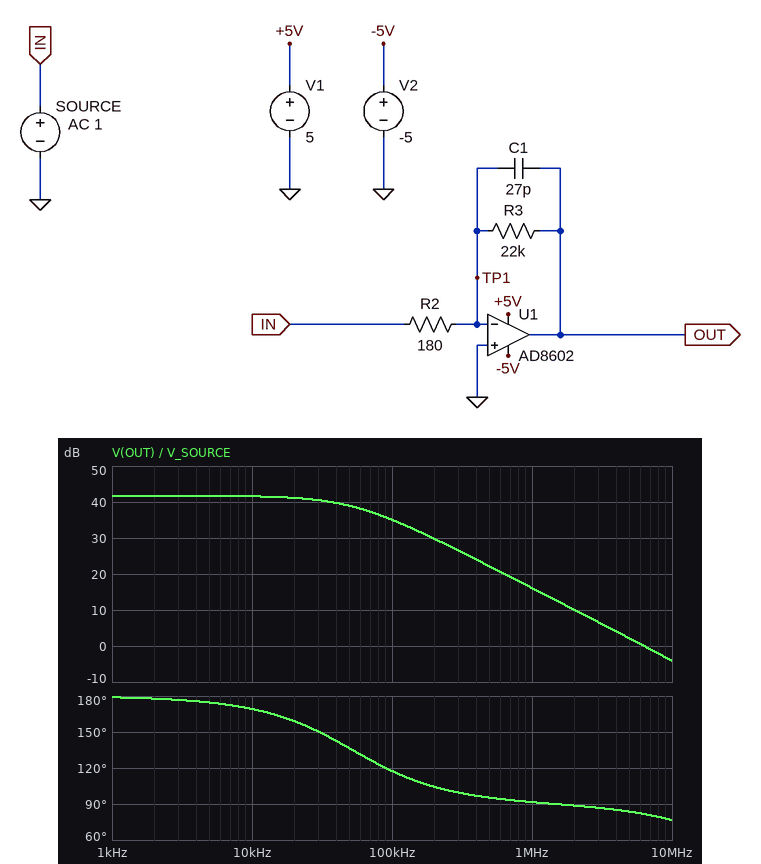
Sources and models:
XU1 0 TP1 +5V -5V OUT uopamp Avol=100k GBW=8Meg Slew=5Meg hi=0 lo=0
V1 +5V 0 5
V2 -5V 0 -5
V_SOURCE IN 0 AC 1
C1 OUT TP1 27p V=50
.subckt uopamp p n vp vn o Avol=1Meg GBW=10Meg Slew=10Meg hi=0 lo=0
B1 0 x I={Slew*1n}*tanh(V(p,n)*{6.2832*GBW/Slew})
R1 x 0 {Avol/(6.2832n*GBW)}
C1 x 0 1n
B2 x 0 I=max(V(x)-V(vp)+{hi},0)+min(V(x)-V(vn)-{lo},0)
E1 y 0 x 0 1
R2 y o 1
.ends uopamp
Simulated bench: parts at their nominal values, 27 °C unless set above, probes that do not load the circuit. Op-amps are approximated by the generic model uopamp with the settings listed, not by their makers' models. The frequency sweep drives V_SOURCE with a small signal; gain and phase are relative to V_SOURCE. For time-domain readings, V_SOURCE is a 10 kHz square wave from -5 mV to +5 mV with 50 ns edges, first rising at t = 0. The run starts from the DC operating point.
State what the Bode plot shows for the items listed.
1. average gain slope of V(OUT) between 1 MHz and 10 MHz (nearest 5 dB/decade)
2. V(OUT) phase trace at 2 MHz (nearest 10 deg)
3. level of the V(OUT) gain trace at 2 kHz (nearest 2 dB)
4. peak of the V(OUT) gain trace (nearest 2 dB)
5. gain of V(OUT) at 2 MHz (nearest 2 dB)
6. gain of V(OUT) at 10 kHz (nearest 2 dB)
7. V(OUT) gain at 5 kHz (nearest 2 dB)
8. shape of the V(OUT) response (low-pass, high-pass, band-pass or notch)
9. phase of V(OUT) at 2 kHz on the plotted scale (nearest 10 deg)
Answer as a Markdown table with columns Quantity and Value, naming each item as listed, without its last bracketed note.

| Quantity | Value |
|---|---|
| average gain slope of V(OUT) between 1 MHz and 10 MHz | -20 dB/decade |
| V(OUT) phase trace at 2 MHz | 90 deg |
| level of the V(OUT) gain trace at 2 kHz | 42 dB |
| peak of the V(OUT) gain trace | 42 dB |
| gain of V(OUT) at 2 MHz | 10 dB |
| gain of V(OUT) at 10 kHz | 42 dB |
| V(OUT) gain at 5 kHz | 42 dB |
| shape of the V(OUT) response | low-pass |
| phase of V(OUT) at 2 kHz on the plotted scale | 180 deg |
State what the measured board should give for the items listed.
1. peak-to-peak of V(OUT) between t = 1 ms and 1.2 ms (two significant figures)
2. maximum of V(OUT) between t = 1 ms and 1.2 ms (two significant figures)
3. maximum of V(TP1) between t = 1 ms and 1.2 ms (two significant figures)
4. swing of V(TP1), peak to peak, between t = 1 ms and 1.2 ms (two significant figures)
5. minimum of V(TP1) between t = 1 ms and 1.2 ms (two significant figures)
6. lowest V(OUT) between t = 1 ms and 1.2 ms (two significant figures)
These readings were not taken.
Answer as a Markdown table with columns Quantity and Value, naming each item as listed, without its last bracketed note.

| Quantity | Value |
|---|---|
| peak-to-peak of V(OUT) between t = 1 ms and 1.2 ms | 1.2 V |
| maximum of V(OUT) between t = 1 ms and 1.2 ms | 610 mV |
| maximum of V(TP1) between t = 1 ms and 1.2 ms | 7.9 mV |
| swing of V(TP1), peak to peak, between t = 1 ms and 1.2 ms | 16 mV |
| minimum of V(TP1) between t = 1 ms and 1.2 ms | -7.9 mV |
| lowest V(OUT) between t = 1 ms and 1.2 ms | -610 mV |
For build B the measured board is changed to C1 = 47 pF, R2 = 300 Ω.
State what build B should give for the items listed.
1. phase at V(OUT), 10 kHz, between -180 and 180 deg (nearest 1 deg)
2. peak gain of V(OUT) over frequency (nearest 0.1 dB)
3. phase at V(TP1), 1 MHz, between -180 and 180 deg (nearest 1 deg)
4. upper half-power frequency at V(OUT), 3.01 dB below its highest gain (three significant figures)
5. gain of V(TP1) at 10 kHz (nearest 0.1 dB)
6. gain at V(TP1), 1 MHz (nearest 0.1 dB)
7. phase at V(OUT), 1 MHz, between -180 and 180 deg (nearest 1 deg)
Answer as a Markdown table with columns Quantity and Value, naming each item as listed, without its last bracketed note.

| Quantity | Value |
|---|---|
| phase at V(OUT), 10 kHz, between -180 and 180 deg | 171 deg |
| peak gain of V(OUT) over frequency | 37.3 dB |
| phase at V(TP1), 1 MHz, between -180 and 180 deg | 1 deg |
| upper half-power frequency at V(OUT), 3.01 dB below its highest gain | 63.6 kHz |
| gain of V(TP1) at 10 kHz | -20.9 dB |
| gain at V(TP1), 1 MHz | -4.7 dB |
| phase at V(OUT), 1 MHz, between -180 and 180 deg | 91 deg |
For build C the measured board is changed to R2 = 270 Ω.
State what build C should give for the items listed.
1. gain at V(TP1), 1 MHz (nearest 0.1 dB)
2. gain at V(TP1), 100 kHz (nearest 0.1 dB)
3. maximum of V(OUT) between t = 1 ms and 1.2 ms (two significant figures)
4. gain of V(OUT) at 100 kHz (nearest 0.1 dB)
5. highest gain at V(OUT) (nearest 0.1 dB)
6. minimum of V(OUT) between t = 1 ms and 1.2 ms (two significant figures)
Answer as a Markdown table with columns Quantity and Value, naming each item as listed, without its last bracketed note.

| Quantity | Value |
|---|---|
| gain at V(TP1), 1 MHz | -2.8 dB |
| gain at V(TP1), 100 kHz | -4.6 dB |
| maximum of V(OUT) between t = 1 ms and 1.2 ms | 410 mV |
| gain of V(OUT) at 100 kHz | 33.5 dB |
| highest gain at V(OUT) | 38.2 dB |
| minimum of V(OUT) between t = 1 ms and 1.2 ms | -410 mV |
